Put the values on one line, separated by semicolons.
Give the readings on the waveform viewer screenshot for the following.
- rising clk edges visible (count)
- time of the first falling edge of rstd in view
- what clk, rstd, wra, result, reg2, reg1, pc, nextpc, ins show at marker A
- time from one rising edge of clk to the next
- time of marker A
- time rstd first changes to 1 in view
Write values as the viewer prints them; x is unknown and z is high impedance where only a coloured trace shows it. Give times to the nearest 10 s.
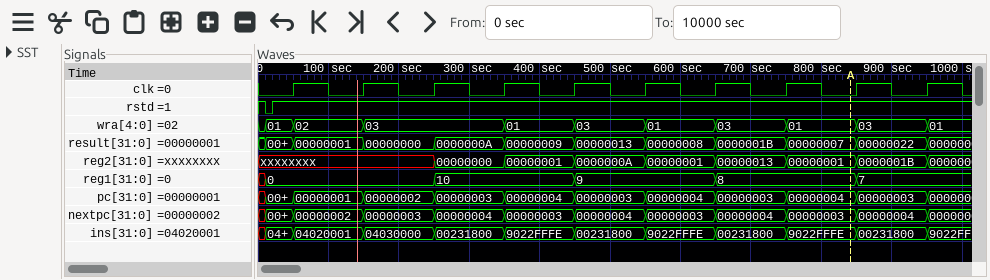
10; 10 s; clk=0, rstd=1, wra=01, result=00000007, reg2=00000001, reg1=8, pc=00000004, nextpc=00000003, ins=9022FFFE; 100 s; 840 s; 20 s
